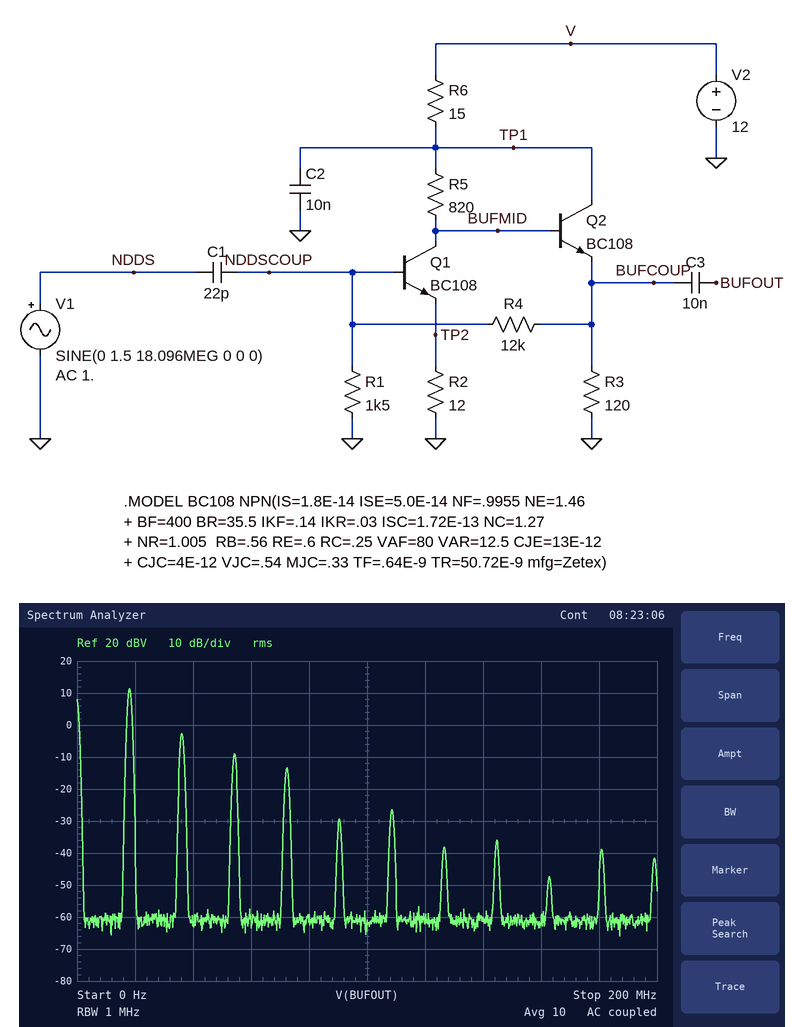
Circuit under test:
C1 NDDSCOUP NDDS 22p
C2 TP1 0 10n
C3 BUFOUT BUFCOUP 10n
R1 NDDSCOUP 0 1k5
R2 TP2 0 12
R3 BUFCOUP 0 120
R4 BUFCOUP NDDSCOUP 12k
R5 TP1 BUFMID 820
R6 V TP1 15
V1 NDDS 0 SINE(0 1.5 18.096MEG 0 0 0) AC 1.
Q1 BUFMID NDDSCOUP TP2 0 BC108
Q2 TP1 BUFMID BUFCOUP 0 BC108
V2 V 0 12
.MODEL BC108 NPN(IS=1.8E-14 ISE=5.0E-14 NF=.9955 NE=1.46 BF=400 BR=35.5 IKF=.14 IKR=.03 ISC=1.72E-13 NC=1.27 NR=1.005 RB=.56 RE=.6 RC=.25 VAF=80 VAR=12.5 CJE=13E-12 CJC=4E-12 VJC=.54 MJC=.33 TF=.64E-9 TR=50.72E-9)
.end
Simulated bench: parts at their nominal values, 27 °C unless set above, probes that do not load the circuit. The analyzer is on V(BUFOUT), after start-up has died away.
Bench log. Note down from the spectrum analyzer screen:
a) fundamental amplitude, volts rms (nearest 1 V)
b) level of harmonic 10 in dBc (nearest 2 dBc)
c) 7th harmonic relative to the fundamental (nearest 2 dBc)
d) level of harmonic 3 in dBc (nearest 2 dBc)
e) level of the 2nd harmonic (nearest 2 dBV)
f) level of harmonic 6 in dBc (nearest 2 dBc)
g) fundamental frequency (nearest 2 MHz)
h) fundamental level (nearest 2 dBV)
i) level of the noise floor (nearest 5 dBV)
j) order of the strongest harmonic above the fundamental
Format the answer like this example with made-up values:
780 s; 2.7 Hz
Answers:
4 V; -50 dBc; -50 dBc; -20 dBc; -2 dBV; -38 dBc; 18 MHz; 12 dBV; -60 dBV; 2
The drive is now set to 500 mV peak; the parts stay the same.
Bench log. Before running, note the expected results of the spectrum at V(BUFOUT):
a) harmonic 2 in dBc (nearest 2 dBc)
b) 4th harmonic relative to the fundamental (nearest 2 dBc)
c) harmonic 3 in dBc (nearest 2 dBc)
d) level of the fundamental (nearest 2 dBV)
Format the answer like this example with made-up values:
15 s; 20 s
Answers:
-24 dBc; -48 dBc; -32 dBc; 6 dBV
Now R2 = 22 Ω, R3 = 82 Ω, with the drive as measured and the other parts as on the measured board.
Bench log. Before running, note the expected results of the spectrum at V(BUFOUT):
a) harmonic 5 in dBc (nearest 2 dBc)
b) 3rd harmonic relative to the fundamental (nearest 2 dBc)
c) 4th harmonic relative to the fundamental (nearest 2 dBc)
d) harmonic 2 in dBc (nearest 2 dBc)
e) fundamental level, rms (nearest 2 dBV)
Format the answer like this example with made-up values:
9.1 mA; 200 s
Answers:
-56 dBc; -28 dBc; -30 dBc; -12 dBc; 10 dBV
